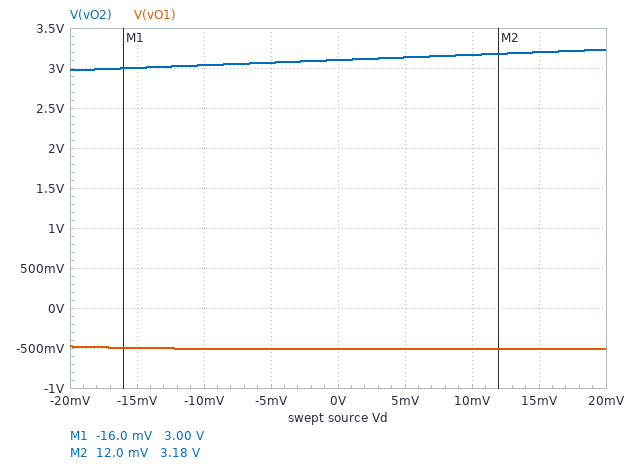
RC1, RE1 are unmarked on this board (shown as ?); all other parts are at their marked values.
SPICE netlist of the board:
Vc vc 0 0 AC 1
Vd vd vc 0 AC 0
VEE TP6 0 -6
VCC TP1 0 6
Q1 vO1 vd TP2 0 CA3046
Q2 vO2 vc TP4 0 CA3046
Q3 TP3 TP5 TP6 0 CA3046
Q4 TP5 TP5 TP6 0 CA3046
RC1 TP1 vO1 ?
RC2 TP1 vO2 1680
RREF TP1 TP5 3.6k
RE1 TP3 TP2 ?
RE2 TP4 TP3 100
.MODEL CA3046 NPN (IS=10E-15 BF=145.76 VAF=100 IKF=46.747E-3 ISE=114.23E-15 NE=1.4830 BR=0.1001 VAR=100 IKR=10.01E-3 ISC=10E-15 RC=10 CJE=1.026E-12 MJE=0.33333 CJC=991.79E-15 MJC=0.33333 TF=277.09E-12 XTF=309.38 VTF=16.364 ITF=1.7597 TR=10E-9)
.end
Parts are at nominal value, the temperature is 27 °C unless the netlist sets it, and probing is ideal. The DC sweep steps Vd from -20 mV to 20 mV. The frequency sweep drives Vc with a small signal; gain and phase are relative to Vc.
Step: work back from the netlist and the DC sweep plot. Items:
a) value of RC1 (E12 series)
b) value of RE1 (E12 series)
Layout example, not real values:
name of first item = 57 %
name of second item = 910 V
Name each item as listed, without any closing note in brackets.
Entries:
value of RC1 = 4.7 kΩ
value of RE1 = 120 Ω
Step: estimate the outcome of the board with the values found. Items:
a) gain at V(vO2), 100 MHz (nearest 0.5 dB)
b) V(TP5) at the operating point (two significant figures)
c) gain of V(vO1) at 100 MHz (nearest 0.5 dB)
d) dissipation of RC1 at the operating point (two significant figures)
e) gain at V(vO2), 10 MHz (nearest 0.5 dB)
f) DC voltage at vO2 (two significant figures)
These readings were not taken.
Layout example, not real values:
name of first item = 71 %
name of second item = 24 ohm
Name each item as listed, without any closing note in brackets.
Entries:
gain at V(vO2), 100 MHz = -13.0 dB
V(TP5) at the operating point = -5.3 V
gain of V(vO1) at 100 MHz = -1.0 dB
dissipation of RC1 at the operating point = 9.0 mW
gain at V(vO2), 10 MHz = -30.0 dB
DC voltage at vO2 = 3.1 V
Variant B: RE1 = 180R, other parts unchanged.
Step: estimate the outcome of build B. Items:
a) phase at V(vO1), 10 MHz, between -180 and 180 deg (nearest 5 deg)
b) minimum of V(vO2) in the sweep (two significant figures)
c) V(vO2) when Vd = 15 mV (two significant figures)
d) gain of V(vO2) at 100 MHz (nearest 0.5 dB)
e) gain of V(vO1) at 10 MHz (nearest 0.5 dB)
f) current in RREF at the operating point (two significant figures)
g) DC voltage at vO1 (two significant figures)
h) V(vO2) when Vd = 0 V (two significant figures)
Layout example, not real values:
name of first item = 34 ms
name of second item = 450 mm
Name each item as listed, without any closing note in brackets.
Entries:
phase at V(vO1), 10 MHz, between -180 and 180 deg = 95 deg
minimum of V(vO2) in the sweep = 2.5 V
V(vO2) when Vd = 15 mV = 2.7 V
gain of V(vO2) at 100 MHz = -12.0 dB
gain of V(vO1) at 10 MHz = -16.5 dB
current in RREF at the operating point = 3.1 mA
DC voltage at vO1 = 420 mV
V(vO2) when Vd = 0 V = 2.6 V
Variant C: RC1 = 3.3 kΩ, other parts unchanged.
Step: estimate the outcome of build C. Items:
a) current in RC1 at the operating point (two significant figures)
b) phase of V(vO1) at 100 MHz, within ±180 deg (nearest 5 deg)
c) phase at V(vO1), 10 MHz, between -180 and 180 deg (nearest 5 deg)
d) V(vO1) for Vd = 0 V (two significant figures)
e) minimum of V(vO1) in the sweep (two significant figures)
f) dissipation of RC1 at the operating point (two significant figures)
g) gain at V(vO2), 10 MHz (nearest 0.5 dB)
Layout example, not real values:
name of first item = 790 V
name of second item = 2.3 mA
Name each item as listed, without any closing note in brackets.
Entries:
current in RC1 at the operating point = 1.5 mA
phase of V(vO1) at 100 MHz, within ±180 deg = 65 deg
phase at V(vO1), 10 MHz, between -180 and 180 deg = 125 deg
V(vO1) for Vd = 0 V = 1.2 V
minimum of V(vO1) in the sweep = 900 mV
dissipation of RC1 at the operating point = 7.1 mW
gain at V(vO2), 10 MHz = -30.5 dB
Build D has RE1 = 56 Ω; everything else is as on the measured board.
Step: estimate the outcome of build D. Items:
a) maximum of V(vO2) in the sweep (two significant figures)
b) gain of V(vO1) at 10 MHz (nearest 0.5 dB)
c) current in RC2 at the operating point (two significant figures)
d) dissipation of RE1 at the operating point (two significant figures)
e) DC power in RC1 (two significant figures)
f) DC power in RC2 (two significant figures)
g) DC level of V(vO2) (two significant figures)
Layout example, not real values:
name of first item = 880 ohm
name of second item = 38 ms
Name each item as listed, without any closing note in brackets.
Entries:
maximum of V(vO2) in the sweep = 4.1 V
gain of V(vO1) at 10 MHz = 0 dB
current in RC2 at the operating point = 1.2 mA
dissipation of RE1 at the operating point = 220 µW
DC power in RC1 = 9.2 mW
DC power in RC2 = 2.6 mW
DC level of V(vO2) = 3.9 V
